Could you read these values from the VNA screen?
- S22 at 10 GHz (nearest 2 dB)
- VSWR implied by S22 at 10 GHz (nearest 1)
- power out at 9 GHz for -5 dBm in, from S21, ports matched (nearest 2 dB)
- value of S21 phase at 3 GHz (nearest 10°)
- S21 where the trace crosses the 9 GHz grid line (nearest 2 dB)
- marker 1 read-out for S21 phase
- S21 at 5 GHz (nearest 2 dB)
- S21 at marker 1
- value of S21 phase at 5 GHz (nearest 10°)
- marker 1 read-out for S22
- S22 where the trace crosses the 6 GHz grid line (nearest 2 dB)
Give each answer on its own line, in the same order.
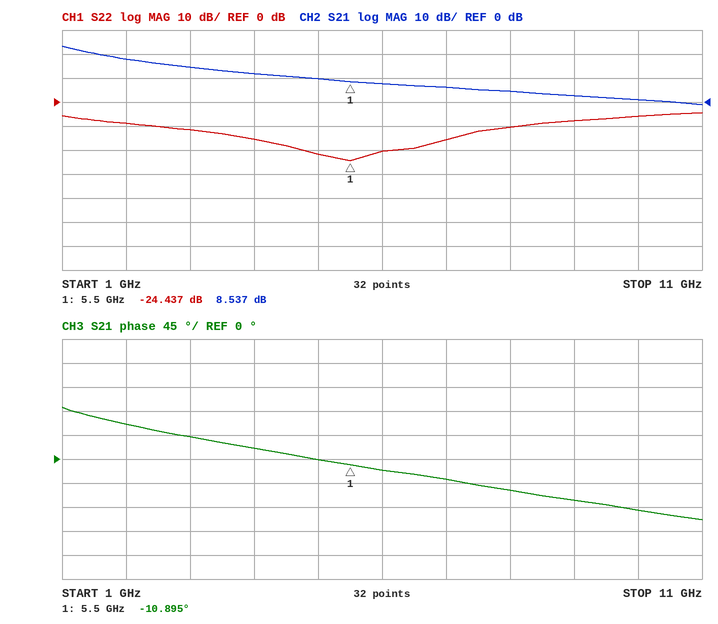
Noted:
-6 dB
3
-2 dBm
40°
2 dB
-10.895°
10 dB
8.537 dB
0°
-24.437 dB
-20 dB
